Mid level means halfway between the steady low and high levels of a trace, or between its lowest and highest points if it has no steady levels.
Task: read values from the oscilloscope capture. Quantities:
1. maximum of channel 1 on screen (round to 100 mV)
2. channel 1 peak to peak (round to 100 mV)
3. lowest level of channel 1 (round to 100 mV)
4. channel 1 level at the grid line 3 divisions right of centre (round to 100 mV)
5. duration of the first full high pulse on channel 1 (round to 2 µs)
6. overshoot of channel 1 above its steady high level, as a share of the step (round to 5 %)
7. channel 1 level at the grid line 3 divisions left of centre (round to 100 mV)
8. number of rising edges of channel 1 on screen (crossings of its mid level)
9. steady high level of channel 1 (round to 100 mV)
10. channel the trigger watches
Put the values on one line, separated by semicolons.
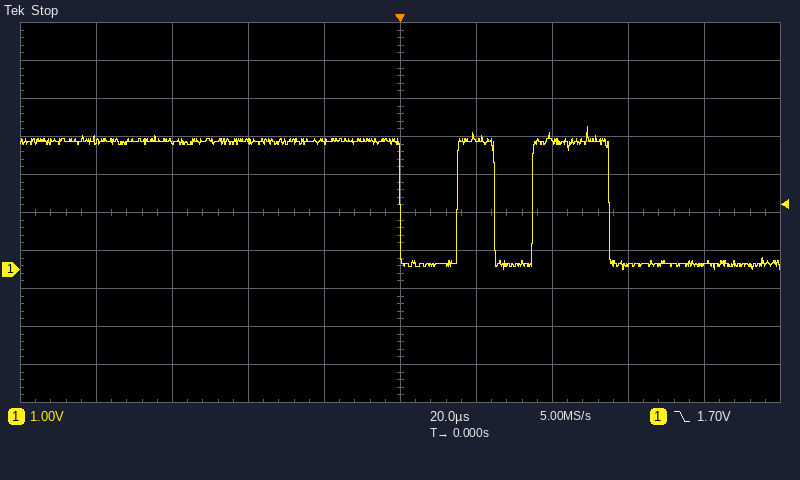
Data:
3.8 V; 3.8 V; 0.0 V; 100 mV; 10 µs; 10 %; 3.4 V; 2; 3.4 V; channel 1
